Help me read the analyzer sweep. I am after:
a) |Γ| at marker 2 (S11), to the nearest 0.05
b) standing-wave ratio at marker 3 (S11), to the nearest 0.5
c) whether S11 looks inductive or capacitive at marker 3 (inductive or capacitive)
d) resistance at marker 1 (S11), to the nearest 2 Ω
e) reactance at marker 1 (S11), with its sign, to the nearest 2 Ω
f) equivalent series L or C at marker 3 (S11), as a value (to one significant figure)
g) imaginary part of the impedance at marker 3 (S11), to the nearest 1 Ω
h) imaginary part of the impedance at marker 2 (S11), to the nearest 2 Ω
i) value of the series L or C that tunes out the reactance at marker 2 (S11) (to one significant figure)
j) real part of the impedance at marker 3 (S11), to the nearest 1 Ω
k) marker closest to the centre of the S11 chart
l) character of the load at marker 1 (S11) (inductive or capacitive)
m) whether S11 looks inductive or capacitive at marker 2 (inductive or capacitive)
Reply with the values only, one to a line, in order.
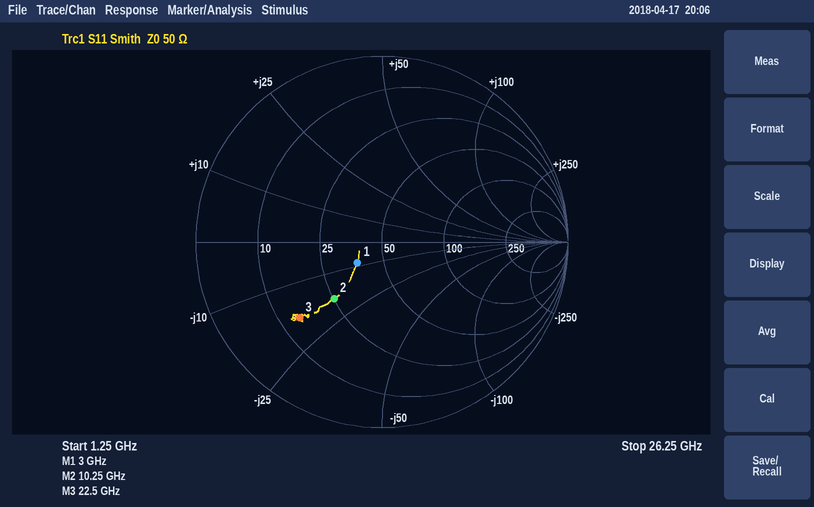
0.40
4.0
capacitive
38 Ω
-8 Ω
400 fF
-18 Ω
-18 Ω
300 pH
14 Ω
marker 1
capacitive
capacitive
